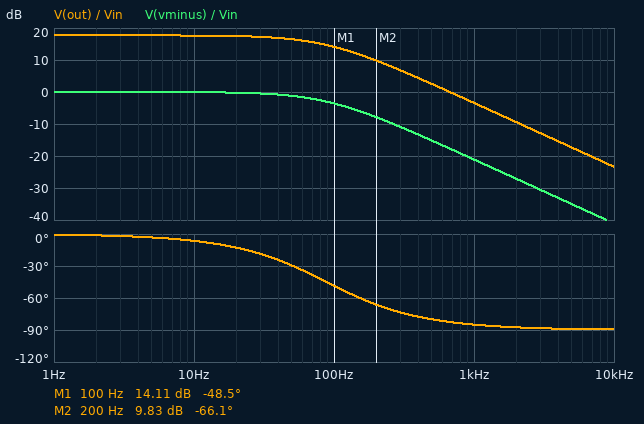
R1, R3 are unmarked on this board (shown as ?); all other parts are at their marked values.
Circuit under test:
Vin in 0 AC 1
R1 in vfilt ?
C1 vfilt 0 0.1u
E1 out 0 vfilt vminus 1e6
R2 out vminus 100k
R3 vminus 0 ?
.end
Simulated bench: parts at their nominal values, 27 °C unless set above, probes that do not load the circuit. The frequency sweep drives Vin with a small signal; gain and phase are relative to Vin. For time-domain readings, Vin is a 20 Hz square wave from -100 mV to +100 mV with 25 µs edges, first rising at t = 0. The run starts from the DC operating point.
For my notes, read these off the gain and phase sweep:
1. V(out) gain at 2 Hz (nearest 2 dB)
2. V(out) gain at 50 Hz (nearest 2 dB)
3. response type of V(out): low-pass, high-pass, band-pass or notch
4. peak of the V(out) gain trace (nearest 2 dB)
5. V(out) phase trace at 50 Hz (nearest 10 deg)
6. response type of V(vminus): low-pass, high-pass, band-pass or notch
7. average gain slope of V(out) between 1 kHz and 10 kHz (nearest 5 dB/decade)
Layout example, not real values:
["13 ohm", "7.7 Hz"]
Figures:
["18 dB", "16 dB", "low-pass", "18 dB", "-30 deg", "low-pass", "-20 dB/decade"]
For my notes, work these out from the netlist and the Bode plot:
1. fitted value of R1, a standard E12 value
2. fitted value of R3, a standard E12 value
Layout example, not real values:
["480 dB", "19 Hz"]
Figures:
["18 kΩ", "15 kΩ"]
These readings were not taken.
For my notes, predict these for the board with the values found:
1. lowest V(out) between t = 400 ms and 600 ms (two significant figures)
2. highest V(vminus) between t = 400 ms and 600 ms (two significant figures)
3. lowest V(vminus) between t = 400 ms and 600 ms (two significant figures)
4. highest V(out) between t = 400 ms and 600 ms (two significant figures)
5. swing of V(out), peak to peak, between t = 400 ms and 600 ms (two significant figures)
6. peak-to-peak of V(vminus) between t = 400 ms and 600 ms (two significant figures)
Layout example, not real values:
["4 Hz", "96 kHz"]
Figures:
["-770 mV", "100 mV", "-100 mV", "770 mV", "1.5 V", "200 mV"]
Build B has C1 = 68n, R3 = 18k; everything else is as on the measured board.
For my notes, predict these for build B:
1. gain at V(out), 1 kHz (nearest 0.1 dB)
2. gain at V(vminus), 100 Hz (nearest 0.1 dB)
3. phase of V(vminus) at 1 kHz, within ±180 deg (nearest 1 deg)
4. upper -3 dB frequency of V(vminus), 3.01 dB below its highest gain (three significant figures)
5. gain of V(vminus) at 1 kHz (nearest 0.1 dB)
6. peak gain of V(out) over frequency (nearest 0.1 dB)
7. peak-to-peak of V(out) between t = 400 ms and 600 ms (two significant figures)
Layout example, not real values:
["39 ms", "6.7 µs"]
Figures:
["-1.5 dB", "-2.0 dB", "-83 deg", "130 Hz", "-17.8 dB", "16.3 dB", "1.3 V"]
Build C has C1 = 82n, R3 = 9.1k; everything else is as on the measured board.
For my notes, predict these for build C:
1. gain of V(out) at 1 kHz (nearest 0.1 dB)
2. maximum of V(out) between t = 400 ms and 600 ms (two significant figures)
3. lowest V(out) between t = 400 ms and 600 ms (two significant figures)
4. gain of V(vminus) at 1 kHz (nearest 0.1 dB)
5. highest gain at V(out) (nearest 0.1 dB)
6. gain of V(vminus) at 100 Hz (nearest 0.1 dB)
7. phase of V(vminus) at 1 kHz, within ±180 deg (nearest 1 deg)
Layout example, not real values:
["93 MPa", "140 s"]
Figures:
["2.2 dB", "1.2 V", "-1.2 V", "-19.4 dB", "21.6 dB", "-2.7 dB", "-84 deg"]
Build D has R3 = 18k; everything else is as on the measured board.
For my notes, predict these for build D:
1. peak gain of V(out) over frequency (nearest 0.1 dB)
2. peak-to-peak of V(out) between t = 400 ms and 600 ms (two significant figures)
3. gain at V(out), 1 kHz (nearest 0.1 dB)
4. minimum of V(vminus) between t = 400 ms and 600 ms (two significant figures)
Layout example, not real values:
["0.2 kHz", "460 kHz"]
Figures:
["16.3 dB", "1.3 V", "-4.8 dB", "-100 mV"]
